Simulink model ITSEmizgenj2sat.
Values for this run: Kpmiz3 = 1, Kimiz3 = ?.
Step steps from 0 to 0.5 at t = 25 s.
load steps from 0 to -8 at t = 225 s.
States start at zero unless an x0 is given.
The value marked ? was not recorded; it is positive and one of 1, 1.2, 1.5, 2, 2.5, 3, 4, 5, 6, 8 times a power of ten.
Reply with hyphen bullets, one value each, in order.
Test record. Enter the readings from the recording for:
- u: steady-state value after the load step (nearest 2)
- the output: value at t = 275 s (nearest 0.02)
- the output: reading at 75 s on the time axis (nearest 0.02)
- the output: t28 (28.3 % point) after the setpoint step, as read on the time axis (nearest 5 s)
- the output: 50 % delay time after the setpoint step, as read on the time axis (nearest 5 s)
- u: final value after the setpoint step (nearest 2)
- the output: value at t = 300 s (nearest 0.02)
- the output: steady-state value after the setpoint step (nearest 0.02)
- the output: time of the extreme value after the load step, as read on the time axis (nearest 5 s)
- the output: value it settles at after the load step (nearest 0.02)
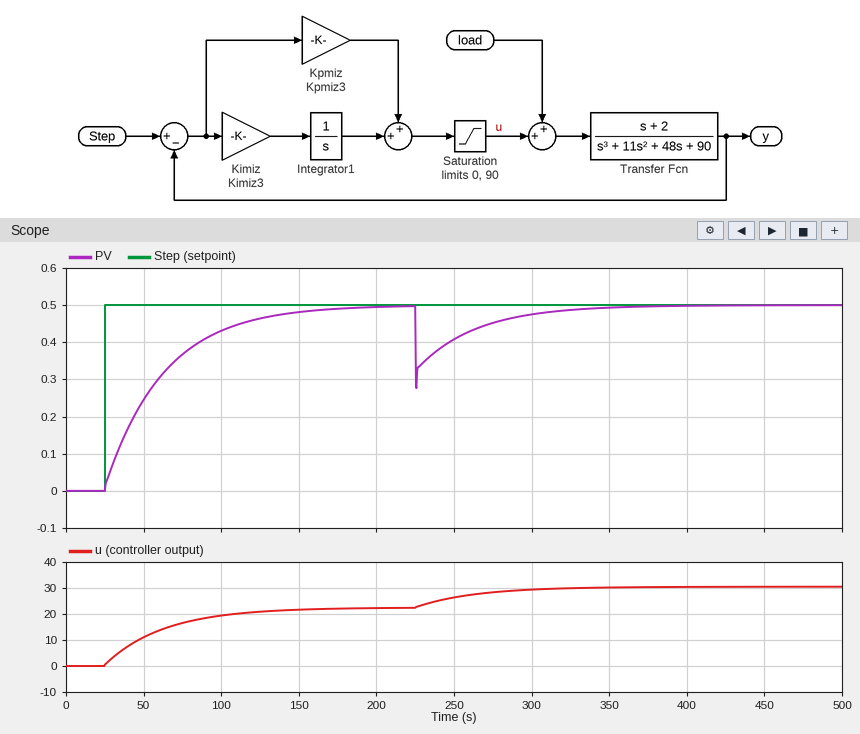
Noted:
- 30
- 0.46
- 0.36
- 35 s
- 50 s
- 22
- 0.48
- 0.50
- 225 s
- 0.50
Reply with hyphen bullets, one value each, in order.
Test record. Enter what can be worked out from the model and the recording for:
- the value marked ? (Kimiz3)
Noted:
- 1.2
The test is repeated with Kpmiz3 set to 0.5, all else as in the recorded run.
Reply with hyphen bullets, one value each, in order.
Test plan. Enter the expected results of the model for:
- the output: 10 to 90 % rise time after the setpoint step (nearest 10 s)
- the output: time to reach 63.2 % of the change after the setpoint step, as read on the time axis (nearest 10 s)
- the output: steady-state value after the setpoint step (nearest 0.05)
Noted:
- 80 s
- 60 s
- 0.50
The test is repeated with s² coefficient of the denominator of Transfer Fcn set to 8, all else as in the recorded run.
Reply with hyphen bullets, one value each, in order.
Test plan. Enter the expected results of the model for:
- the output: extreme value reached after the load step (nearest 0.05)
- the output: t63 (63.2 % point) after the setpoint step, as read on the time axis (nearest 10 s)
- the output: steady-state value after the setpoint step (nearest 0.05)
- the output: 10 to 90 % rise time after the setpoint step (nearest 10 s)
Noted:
- 0.25
- 60 s
- 0.50
- 80 s
